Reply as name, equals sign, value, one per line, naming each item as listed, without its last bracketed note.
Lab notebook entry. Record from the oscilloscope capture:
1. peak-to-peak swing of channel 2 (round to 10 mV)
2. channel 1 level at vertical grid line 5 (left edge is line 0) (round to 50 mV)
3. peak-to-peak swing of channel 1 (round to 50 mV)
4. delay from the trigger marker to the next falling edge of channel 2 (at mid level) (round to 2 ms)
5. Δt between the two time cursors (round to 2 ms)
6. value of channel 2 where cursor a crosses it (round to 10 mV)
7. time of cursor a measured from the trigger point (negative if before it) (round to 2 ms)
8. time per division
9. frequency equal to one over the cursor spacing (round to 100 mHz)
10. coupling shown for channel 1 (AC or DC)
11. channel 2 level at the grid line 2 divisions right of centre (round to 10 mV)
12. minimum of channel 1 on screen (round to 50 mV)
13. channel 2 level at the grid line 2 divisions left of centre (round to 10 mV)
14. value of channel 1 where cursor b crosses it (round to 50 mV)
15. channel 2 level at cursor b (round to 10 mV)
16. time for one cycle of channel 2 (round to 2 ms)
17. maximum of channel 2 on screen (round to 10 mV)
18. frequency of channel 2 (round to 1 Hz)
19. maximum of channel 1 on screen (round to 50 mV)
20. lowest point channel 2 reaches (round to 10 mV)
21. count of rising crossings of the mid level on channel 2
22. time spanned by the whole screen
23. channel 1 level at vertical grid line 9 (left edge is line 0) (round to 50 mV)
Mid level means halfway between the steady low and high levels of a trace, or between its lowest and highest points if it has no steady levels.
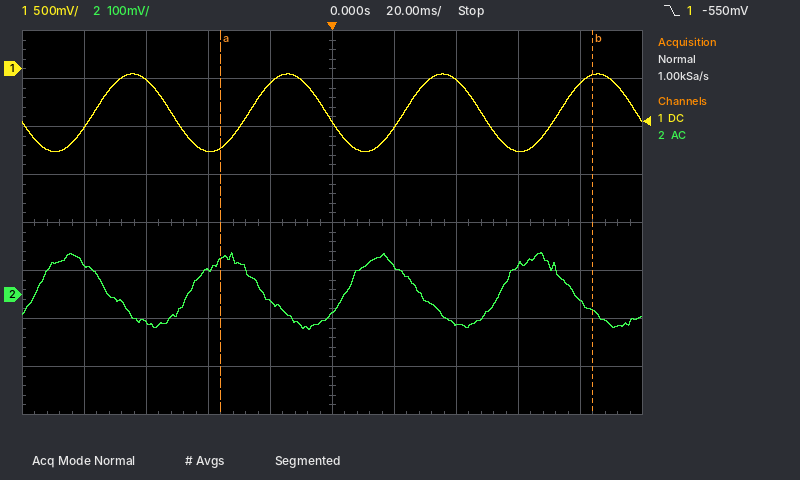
peak-to-peak swing of channel 2 = 160 mV
channel 1 level at vertical grid line 5 (left edge is line 0) = -550 mV
peak-to-peak swing of channel 1 = 800 mV
delay from the trigger marker to the next falling edge of channel 2 (at mid level) = 28 ms
Δt between the two time cursors = 120 ms
value of channel 2 where cursor a crosses it = 70 mV
time of cursor a measured from the trigger point (negative if before it) = -36 ms
time per division = 20 ms
frequency equal to one over the cursor spacing = 8.3 Hz
coupling shown for channel 1 = DC
channel 2 level at the grid line 2 divisions right of centre = -60 mV
minimum of channel 1 on screen = -850 mV
channel 2 level at the grid line 2 divisions left of centre = 50 mV
value of channel 1 where cursor b crosses it = -50 mV
channel 2 level at cursor b = -30 mV
time for one cycle of channel 2 = 50 ms
maximum of channel 2 on screen = 90 mV
frequency of channel 2 = 20 Hz
maximum of channel 1 on screen = -50 mV
lowest point channel 2 reaches = -70 mV
count of rising crossings of the mid level on channel 2 = 4
time spanned by the whole screen = 200 ms
channel 1 level at vertical grid line 9 (left edge is line 0) = -150 mV
